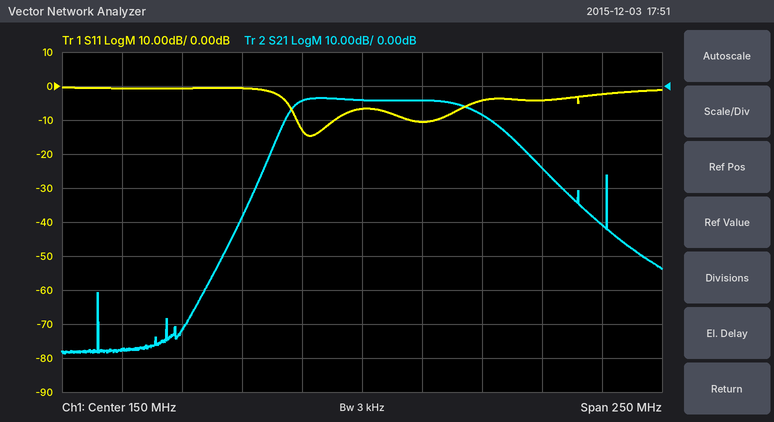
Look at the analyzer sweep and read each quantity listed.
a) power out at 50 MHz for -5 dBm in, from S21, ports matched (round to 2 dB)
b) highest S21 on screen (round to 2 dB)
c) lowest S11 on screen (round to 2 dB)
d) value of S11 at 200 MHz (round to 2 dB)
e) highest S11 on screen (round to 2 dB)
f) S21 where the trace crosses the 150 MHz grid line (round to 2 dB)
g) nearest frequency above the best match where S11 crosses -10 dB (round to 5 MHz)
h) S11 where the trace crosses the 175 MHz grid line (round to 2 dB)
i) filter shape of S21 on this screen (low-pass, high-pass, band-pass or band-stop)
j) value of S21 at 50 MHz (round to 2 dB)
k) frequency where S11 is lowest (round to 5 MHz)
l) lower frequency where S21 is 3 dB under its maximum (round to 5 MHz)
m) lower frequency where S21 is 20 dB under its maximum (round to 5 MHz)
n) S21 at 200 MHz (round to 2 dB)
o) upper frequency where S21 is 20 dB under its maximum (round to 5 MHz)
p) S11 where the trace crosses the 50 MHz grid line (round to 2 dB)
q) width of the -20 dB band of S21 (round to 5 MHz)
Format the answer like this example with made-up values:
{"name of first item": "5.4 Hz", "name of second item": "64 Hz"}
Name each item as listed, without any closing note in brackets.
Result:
{"power out at 50 MHz for -5 dBm in, from S21, ports matched": "-82 dBm", "highest S21 on screen": "-4 dB", "lowest S11 on screen": "-14 dB", "value of S11 at 200 MHz": "-4 dB", "highest S11 on screen": "0 dB", "S21 where the trace crosses the 150 MHz grid line": "-4 dB", "nearest frequency above the best match where S11 crosses -10 dB": "140 MHz", "S11 where the trace crosses the 175 MHz grid line": "-10 dB", "filter shape of S21 on this screen": "band-pass", "value of S21 at 50 MHz": "-78 dB", "frequency where S11 is lowest": "130 MHz", "lower frequency where S21 is 3 dB under its maximum": "120 MHz", "lower frequency where S21 is 20 dB under its maximum": "110 MHz", "S21 at 200 MHz": "-8 dB", "upper frequency where S21 is 20 dB under its maximum": "225 MHz", "S11 where the trace crosses the 50 MHz grid line": "0 dB", "width of the -20 dB band of S21": "115 MHz"}
